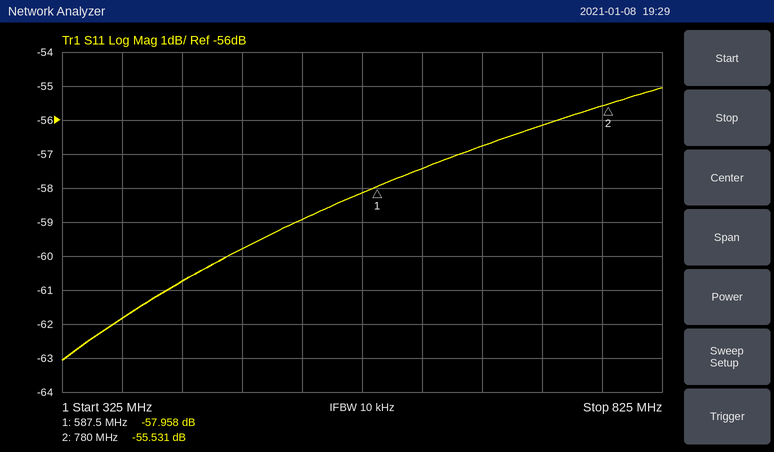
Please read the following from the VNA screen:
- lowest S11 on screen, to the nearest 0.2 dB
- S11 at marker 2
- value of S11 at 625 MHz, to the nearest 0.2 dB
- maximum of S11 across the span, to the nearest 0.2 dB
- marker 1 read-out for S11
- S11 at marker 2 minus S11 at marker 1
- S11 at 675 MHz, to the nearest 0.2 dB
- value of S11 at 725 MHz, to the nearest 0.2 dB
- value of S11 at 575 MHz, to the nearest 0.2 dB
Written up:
-63.0 dB
-55.531 dB
-57.4 dB
-55.0 dB
-57.958 dB
2.427 dB
-56.8 dB
-56.2 dB
-58.2 dB
